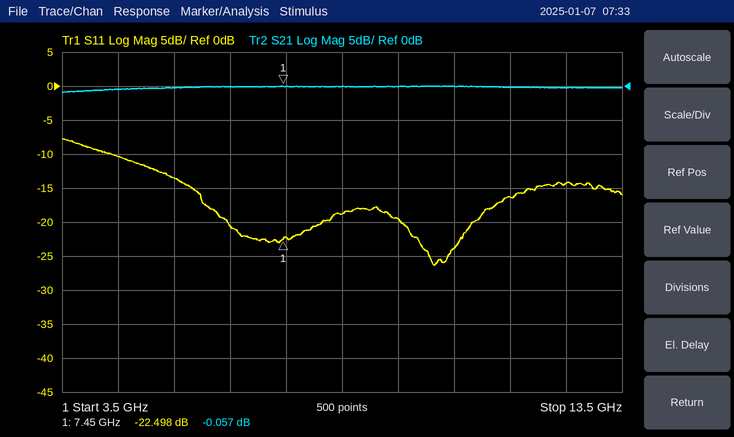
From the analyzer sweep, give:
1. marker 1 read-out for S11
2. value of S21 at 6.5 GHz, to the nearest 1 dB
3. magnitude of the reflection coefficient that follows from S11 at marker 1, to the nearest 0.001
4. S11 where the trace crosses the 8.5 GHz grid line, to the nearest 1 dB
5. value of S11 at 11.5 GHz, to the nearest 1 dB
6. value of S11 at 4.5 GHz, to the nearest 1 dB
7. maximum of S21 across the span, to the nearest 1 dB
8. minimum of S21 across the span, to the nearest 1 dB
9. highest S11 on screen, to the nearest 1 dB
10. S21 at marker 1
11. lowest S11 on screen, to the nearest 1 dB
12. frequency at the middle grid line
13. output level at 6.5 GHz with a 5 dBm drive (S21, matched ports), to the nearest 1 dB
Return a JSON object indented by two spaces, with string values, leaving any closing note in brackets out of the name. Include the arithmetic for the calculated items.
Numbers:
{
  "marker 1 read-out for S11": "-22.498 dB",
  "value of S21 at 6.5 GHz, to the nearest 1 dB": "0 dB",
  "magnitude of the reflection coefficient that follows from S11 at marker 1, to the nearest 0.001": "10^(-22.498/20) ≈ 0.075",
  "S11 where the trace crosses the 8.5 GHz grid line, to the nearest 1 dB": "-19 dB",
  "value of S11 at 11.5 GHz, to the nearest 1 dB": "-16 dB",
  "value of S11 at 4.5 GHz, to the nearest 1 dB": "-10 dB",
  "maximum of S21 across the span, to the nearest 1 dB": "0 dB",
  "minimum of S21 across the span, to the nearest 1 dB": "-1 dB",
  "highest S11 on screen, to the nearest 1 dB": "-8 dB",
  "S21 at marker 1": "-0.057 dB",
  "lowest S11 on screen, to the nearest 1 dB": "-26 dB",
  "frequency at the middle grid line": "8.5 GHz",
  "output level at 6.5 GHz with a 5 dBm drive (S21, matched ports), to the nearest 1 dB": "5 dBm + (0 dB) = 5 dBm"
}
